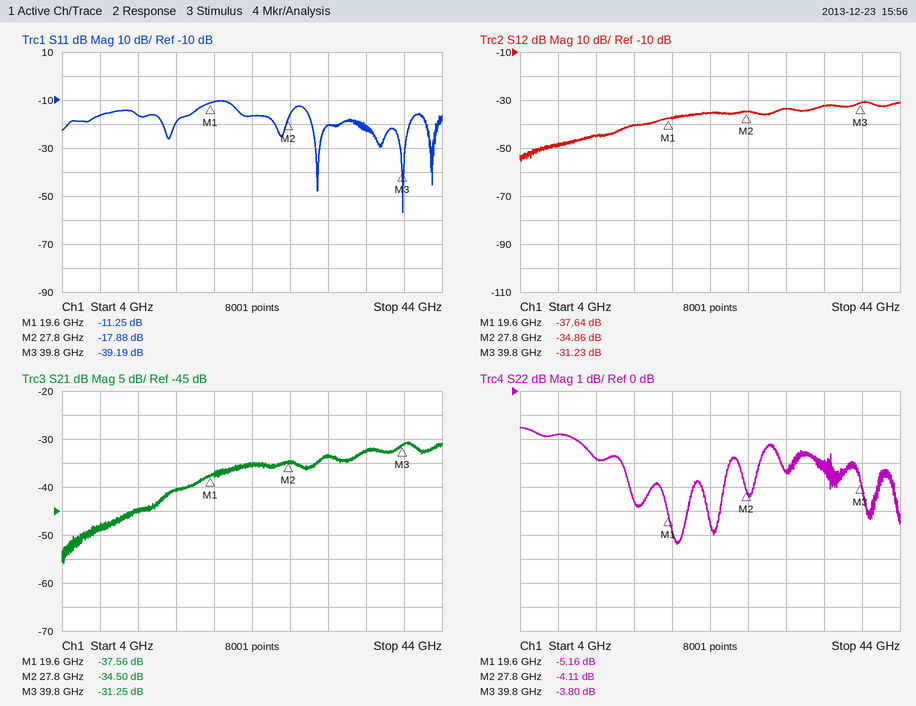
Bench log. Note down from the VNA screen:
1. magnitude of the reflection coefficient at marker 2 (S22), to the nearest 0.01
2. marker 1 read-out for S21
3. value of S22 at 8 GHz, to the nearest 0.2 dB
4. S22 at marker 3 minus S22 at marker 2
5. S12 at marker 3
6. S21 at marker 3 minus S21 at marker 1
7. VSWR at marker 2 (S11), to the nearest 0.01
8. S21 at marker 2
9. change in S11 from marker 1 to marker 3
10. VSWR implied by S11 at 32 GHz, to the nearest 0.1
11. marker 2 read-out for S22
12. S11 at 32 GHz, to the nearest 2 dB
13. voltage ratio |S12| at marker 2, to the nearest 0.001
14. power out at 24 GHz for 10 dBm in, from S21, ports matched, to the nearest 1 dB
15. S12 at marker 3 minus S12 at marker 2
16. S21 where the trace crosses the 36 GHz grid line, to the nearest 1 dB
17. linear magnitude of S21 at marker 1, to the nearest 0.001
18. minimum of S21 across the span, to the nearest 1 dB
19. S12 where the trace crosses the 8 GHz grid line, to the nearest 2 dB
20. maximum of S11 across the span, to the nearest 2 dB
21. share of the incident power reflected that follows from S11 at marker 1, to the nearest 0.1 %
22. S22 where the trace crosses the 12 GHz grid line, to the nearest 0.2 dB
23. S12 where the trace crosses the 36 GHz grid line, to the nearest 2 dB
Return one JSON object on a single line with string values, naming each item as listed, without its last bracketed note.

{"magnitude of the reflection coefficient at marker 2 (S22), to the nearest 0.01": "0.62", "marker 1 read-out for S21": "-37.56 dB", "value of S22 at 8 GHz, to the nearest 0.2 dB": "-1.8 dB", "S22 at marker 3 minus S22 at marker 2": "0.31 dB", "S12 at marker 3": "-31.23 dB", "S21 at marker 3 minus S21 at marker 1": "6.31 dB", "VSWR at marker 2 (S11), to the nearest 0.01": "1.29", "S21 at marker 2": "-34.50 dB", "change in S11 from marker 1 to marker 3": "-27.94 dB", "VSWR implied by S11 at 32 GHz, to the nearest 0.1": "1.2", "marker 2 read-out for S22": "-4.11 dB", "S11 at 32 GHz, to the nearest 2 dB": "-20 dB", "voltage ratio |S12| at marker 2, to the nearest 0.001": "0.018", "power out at 24 GHz for 10 dBm in, from S21, ports matched, to the nearest 1 dB": "-25 dBm", "S12 at marker 3 minus S12 at marker 2": "3.63 dB", "S21 where the trace crosses the 36 GHz grid line, to the nearest 1 dB": "-32 dB", "linear magnitude of S21 at marker 1, to the nearest 0.001": "0.013", "minimum of S21 across the span, to the nearest 1 dB": "-56 dB", "S12 where the trace crosses the 8 GHz grid line, to the nearest 2 dB": "-48 dB", "maximum of S11 across the span, to the nearest 2 dB": "-10 dB", "share of the incident power reflected that follows from S11 at marker 1, to the nearest 0.1 %": "7.5 %", "S22 where the trace crosses the 12 GHz grid line, to the nearest 0.2 dB": "-2.8 dB", "S12 where the trace crosses the 36 GHz grid line, to the nearest 2 dB": "-32 dB"}
